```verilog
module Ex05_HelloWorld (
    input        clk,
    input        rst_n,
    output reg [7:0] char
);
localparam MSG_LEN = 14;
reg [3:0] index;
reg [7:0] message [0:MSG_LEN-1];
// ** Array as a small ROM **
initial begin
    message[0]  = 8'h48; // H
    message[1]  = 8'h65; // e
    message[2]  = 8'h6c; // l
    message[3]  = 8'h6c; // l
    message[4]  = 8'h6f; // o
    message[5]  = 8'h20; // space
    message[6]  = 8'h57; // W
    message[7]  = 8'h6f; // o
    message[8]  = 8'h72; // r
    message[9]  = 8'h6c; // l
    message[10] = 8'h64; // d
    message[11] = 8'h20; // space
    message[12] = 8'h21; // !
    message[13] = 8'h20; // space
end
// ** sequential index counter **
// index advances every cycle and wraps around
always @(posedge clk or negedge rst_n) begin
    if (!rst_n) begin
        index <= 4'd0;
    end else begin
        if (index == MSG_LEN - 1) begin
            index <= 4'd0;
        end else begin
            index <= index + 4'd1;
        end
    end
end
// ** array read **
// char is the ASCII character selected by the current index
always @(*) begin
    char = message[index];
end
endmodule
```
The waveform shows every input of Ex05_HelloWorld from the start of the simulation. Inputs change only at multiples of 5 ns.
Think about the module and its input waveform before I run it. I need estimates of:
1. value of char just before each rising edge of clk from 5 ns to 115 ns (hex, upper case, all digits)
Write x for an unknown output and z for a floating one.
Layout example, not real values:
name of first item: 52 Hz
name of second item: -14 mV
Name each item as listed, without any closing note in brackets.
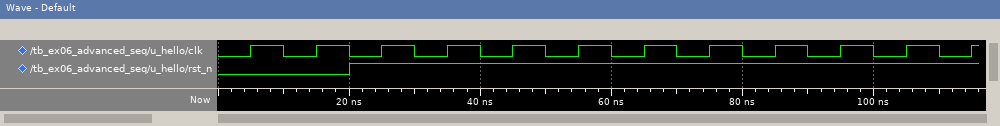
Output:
value of char just before each rising edge of clk from 5 ns to 115 ns: 48, 48, 48, 65, 6C, 6C, 6F, 20, 57, 6F, 72, 6C
